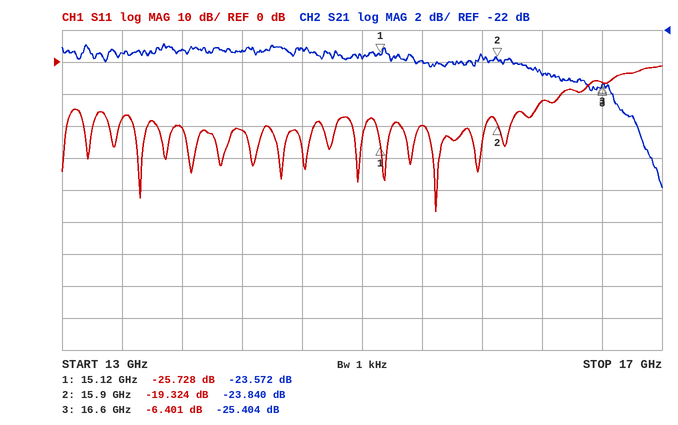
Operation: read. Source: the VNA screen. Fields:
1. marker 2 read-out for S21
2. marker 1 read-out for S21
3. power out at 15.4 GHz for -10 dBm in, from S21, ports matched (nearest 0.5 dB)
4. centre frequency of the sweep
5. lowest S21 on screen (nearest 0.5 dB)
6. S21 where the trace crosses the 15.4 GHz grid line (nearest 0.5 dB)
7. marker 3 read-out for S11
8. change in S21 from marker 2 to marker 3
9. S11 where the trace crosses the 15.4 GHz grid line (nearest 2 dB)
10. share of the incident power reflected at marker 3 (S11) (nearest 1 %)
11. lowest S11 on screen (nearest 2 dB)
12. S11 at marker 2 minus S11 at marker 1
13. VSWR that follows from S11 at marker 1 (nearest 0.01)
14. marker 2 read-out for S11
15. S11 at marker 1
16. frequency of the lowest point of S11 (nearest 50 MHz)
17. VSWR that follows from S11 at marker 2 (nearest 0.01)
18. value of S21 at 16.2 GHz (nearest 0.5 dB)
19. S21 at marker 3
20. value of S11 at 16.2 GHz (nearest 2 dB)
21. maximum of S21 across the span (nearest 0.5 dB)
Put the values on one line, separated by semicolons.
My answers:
-23.840 dB; -23.572 dB; -34.0 dBm; 15 GHz; -32.0 dB; -24.0 dB; -6.401 dB; -1.564 dB; -20 dB; 23 %; -46 dB; 6.404 dB; 1.11; -19.324 dB; -25.728 dB; 15.50 GHz; 1.24; -25.0 dB; -25.404 dB; -12 dB; -23.0 dB
